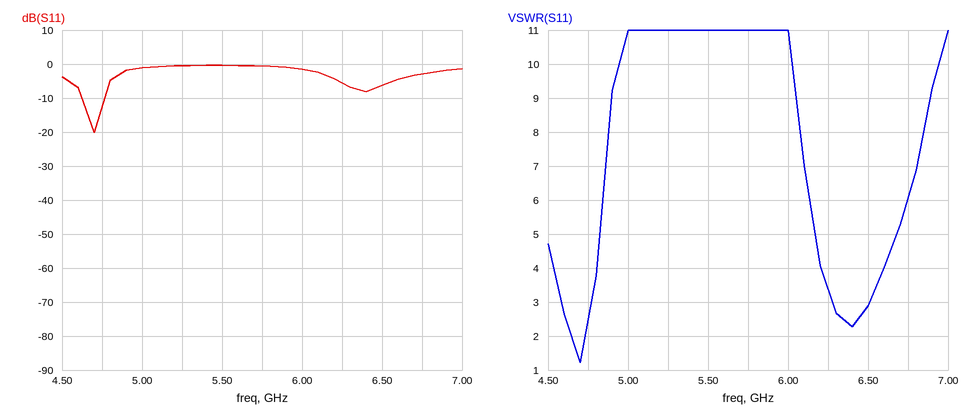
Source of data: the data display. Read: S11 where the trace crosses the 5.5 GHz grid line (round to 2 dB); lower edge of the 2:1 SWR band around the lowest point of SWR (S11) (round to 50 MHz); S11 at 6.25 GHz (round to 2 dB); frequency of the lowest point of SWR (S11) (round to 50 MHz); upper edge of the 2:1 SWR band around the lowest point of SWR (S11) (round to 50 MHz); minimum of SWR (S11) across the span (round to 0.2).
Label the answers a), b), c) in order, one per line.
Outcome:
a) 0 dB
b) 4.65 GHz
c) -6 dB
d) 4.70 GHz
e) 4.75 GHz
f) 1.2
